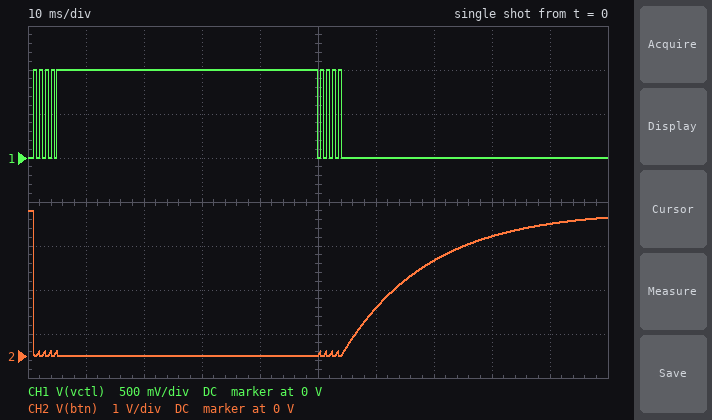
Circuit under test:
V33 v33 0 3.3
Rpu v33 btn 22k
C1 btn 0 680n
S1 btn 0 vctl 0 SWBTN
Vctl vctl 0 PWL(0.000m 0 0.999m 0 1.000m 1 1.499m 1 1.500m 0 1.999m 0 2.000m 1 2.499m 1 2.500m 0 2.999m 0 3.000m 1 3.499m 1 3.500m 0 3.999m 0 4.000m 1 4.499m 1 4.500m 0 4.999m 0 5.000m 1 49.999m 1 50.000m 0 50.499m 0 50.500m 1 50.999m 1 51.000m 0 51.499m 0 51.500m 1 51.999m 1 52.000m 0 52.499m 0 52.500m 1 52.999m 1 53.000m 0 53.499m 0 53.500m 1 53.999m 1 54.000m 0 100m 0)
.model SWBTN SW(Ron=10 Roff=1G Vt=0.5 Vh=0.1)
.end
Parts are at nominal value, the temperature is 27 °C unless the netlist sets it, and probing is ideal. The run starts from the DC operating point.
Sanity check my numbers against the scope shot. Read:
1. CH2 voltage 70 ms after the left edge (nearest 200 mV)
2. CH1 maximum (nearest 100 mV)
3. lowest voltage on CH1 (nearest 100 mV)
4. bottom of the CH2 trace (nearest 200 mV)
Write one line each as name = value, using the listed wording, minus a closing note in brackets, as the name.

CH2 voltage 70 ms after the left edge = 2.2 V
CH1 maximum = 1.0 V
lowest voltage on CH1 = 0 V
bottom of the CH2 trace = 0 V
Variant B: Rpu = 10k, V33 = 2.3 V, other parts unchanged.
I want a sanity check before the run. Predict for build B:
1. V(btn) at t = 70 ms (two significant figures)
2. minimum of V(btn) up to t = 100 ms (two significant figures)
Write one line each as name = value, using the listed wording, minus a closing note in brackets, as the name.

V(btn) at t = 70 ms = 2.1 V
minimum of V(btn) up to t = 100 ms = 2.3 mV
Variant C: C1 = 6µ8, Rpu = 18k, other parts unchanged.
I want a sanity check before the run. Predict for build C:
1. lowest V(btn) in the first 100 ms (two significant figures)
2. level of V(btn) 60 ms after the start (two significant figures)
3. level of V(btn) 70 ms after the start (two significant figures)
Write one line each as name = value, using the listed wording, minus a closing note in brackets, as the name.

lowest V(btn) in the first 100 ms = 1.8 mV
level of V(btn) 60 ms after the start = 160 mV
level of V(btn) 70 ms after the start = 410 mV
